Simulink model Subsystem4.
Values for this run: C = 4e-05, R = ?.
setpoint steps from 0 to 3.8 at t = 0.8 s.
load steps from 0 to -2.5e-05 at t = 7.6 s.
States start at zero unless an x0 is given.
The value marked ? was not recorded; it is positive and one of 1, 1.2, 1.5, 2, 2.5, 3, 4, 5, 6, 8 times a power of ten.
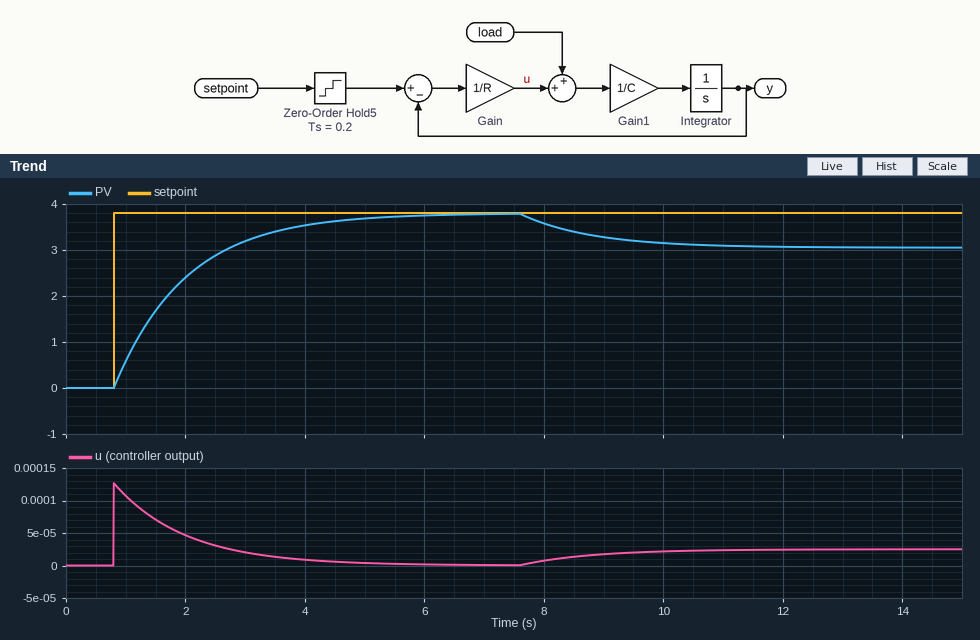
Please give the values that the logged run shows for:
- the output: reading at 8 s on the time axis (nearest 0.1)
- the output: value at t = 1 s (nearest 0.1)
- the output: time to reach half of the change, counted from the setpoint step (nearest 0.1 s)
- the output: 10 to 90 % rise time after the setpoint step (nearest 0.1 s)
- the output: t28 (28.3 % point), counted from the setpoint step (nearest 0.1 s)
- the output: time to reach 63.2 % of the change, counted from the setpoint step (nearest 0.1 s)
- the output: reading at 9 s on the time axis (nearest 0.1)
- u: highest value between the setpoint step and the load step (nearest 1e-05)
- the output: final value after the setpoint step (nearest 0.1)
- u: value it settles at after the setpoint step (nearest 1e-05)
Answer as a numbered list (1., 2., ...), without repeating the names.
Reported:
1. 3.6
2. 0.6
3. 0.8 s
4. 2.6 s
5. 0.4 s
6. 1.2 s
7. 3.3
8. 0.00013
9. 3.8
10. 0.00000
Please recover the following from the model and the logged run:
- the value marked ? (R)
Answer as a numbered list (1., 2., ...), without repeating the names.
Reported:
1. 30000
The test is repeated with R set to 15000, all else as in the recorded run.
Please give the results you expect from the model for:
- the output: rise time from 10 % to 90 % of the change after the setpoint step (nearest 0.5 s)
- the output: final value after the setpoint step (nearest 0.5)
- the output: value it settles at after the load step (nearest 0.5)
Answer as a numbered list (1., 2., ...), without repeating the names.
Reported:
1. 1.5 s
2. 4.0
3. 3.5
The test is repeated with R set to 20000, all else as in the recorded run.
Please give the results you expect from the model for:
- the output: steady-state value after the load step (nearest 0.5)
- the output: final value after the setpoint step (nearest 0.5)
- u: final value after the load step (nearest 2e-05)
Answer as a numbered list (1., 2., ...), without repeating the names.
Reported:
1. 3.5
2. 4.0
3. 0.00002
